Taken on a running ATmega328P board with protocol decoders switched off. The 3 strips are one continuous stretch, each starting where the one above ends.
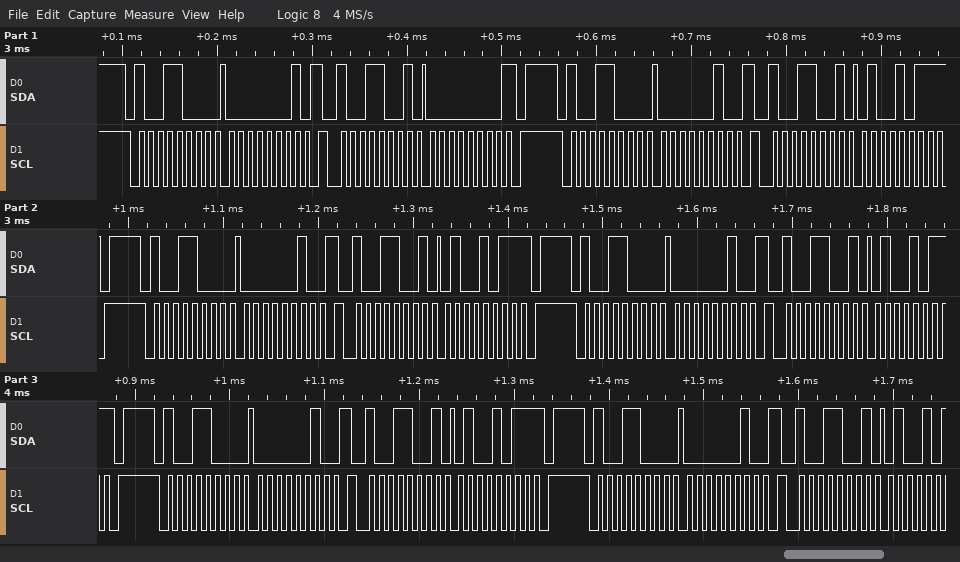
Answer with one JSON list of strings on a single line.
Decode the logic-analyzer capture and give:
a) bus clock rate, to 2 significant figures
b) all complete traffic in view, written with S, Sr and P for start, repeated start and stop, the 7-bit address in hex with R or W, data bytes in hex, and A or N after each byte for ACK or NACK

["100 kHz", "S 4CW A 01 A Sr 4CR A 00 N P S 4CW A 02 A Sr 4CR A 4B N P S 4CW A 02 A Sr 4CR A 4B N P S 4CW A 02 A Sr 4CR A 4B N P S 4CW A 02 A Sr 4CR A 4B N P S 4CW A 02 A Sr 4CR A"]
